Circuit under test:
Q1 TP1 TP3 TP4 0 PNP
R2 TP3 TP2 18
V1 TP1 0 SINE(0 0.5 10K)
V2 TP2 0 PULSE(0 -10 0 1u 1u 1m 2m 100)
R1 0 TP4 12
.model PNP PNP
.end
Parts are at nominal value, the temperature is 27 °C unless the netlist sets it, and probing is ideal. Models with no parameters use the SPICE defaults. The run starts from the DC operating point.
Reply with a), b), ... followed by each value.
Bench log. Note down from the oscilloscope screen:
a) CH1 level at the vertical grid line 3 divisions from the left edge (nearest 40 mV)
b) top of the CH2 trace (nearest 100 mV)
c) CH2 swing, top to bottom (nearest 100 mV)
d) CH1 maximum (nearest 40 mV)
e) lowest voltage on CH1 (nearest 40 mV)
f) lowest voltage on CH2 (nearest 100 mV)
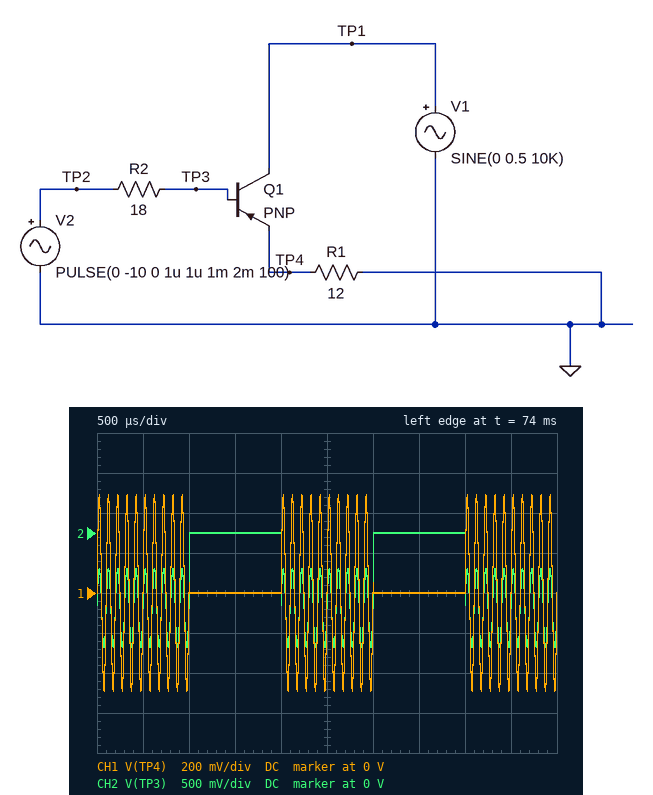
a) 0 V
b) 0 V
c) 1.4 V
d) 480 mV
e) -480 mV
f) -1.4 V
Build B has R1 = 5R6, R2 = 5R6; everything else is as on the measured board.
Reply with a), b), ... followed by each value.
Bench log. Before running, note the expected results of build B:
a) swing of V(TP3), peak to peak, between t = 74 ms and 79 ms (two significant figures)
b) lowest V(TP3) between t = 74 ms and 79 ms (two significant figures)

a) 1.5 V
b) -1.5 V
